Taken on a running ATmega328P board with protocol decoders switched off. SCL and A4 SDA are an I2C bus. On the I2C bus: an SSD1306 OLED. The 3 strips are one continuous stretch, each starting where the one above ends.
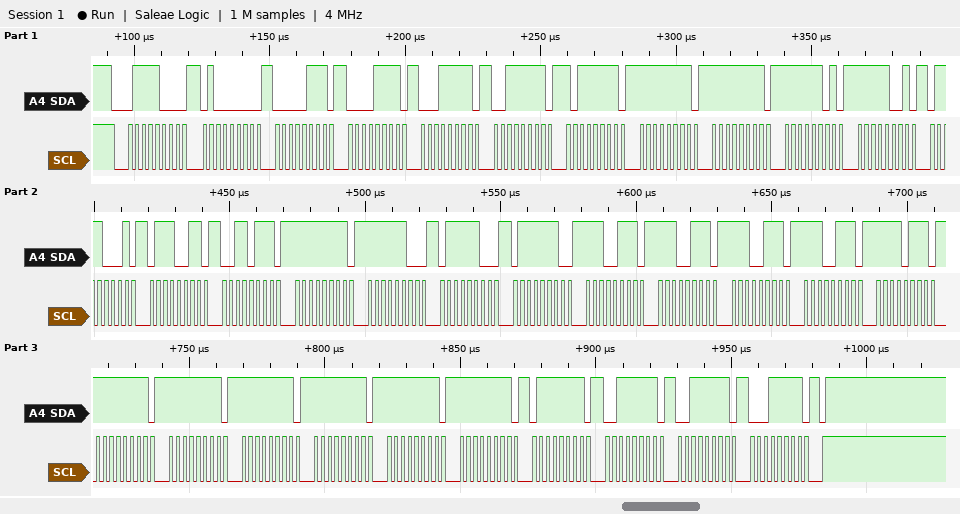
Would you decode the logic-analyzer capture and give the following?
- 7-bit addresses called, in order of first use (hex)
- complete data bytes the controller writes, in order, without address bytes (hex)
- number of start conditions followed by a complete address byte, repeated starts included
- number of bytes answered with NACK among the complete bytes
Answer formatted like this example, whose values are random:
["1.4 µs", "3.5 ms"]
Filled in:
["0x3C", "40 07 0F 1F 3F BF FF FF FD F9 71 73 37 FF FC 7C 7E E7 E7 E7 E7 F7 FF FF FF FF FF FF 7F 3F 3F 1F", "1", "0"]
